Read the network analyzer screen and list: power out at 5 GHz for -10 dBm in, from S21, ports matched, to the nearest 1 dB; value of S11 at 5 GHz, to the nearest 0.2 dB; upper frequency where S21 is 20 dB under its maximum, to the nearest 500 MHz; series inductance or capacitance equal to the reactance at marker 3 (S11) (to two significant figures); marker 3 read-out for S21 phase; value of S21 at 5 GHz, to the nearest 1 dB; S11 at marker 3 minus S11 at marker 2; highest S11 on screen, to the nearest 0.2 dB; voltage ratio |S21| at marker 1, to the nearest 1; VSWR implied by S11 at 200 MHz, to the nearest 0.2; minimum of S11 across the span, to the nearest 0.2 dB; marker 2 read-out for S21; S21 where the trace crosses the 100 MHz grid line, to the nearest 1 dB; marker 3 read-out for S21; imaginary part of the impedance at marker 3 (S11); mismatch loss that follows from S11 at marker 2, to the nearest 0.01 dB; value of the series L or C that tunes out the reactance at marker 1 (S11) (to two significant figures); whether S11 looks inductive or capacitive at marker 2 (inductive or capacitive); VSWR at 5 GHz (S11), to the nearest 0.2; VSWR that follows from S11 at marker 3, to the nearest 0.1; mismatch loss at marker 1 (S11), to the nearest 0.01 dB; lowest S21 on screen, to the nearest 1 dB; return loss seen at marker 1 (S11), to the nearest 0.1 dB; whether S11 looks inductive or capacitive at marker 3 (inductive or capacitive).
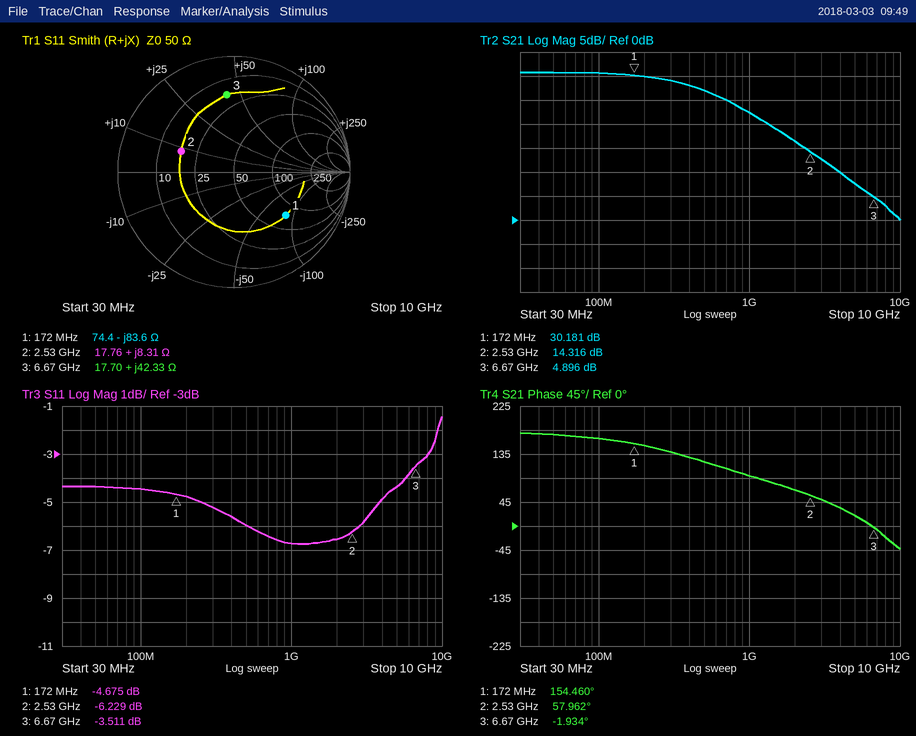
-2 dBm
-4.4 dB
3.5 GHz
1.0 nH
-1.934°
8 dB
2.718 dB
-1.4 dB
32
3.8
-6.8 dB
14.316 dB
31 dB
4.896 dB
+42.33 Ω
1.18 dB
77 nH
inductive
4.0
5.0
1.81 dB
0 dB
4.7 dB
inductive
